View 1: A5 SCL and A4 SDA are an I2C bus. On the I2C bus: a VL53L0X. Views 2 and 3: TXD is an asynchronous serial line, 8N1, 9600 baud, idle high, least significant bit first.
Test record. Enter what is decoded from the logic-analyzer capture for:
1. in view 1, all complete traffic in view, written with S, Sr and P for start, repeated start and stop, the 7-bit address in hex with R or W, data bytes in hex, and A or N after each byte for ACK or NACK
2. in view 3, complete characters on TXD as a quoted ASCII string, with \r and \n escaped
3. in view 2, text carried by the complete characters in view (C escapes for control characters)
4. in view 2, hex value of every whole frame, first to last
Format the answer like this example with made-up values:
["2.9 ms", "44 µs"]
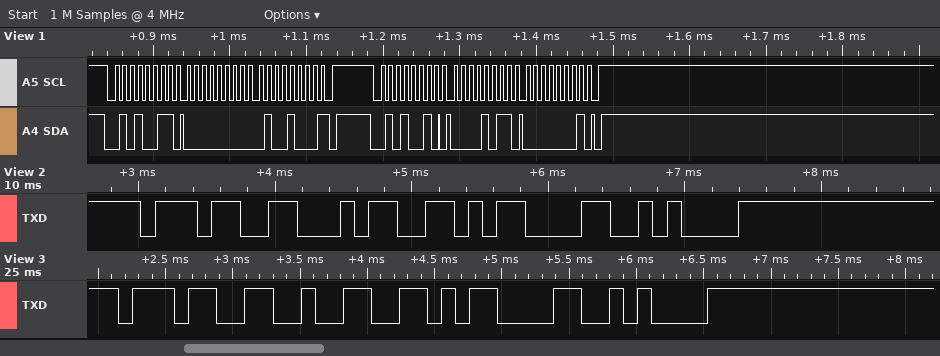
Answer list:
["S 29R A 00 A 48 N P S 29W A 0B A 01 A P", "\"72\\r\\n\"", "\"74\\r\\n\"", "37 34 0D 0A"]
